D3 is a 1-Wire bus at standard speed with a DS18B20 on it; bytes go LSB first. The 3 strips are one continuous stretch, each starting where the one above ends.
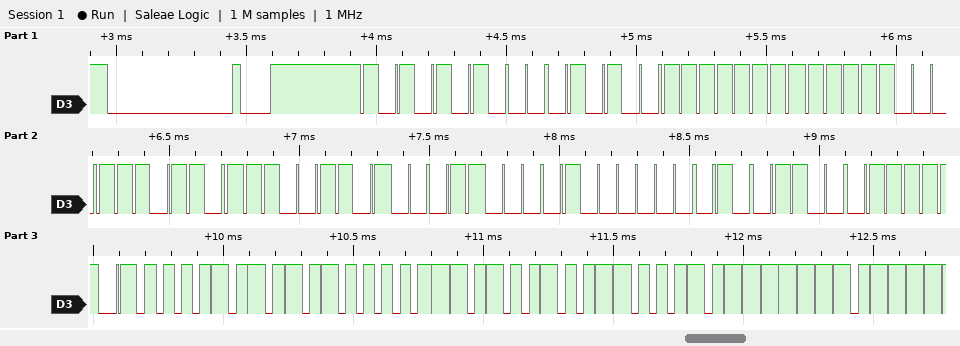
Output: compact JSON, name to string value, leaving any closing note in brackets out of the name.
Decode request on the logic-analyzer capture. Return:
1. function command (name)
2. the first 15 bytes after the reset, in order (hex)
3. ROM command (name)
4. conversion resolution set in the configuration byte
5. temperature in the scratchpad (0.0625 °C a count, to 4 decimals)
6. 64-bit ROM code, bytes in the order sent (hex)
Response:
{"function command": "Read Scratchpad", "the first 15 bytes after the reset, in order": "55 28 FF 1F B7 B3 18 02 32 BE 50 05 4B 46 7F", "ROM command": "Match ROM", "conversion resolution set in the configuration byte": "12 bits", "temperature in the scratchpad": "85.0000 °C", "64-bit ROM code, bytes in the order sent": "28 FF 1F B7 B3 18 02 32"}
